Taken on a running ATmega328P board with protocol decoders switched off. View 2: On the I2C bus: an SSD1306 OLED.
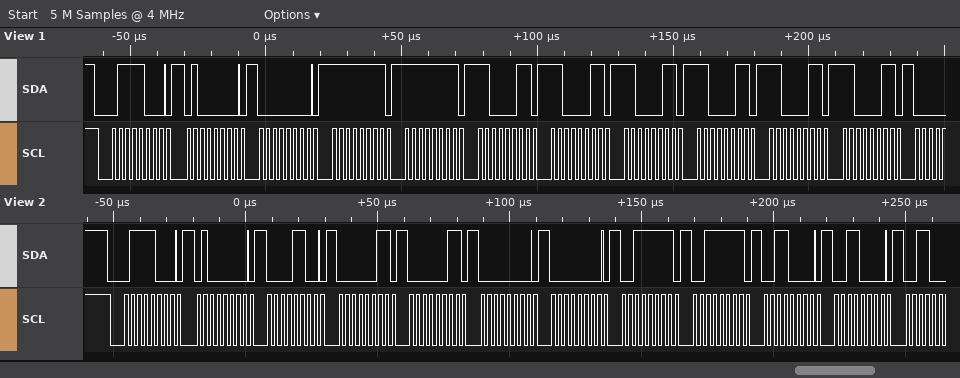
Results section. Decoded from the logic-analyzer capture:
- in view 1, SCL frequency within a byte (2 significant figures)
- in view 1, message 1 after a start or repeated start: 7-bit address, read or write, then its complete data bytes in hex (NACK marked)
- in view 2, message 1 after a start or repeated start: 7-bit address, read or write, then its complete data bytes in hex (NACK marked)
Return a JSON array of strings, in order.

["400 kHz", "0x3C write: 40 00 FF FF C3 C3 C3 C3 C3 C3", "0x3C write: 40 0C 03 03 00 00 3F 3F 30 30"]
